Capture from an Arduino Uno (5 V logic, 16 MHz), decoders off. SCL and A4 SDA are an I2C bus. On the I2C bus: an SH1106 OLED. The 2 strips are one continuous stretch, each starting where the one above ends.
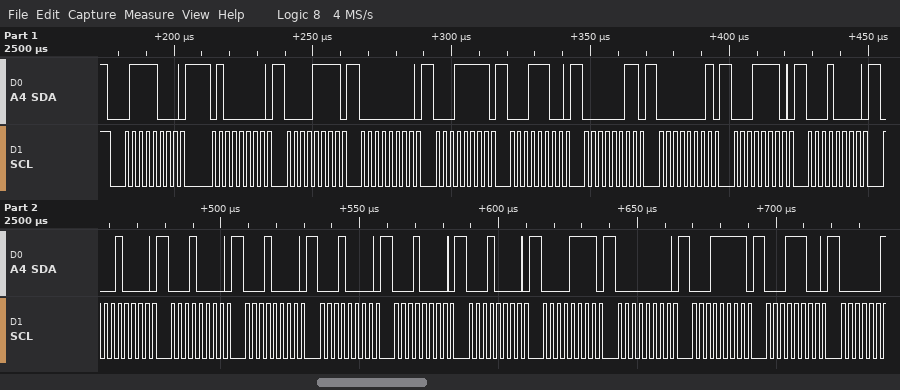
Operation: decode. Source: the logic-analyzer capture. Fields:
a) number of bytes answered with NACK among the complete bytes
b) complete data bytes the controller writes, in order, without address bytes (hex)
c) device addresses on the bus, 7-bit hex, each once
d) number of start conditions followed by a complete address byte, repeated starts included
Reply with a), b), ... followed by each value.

a) 0
b) 40 0F 00 1F 1C 03 01 1E 10 10 10 10 10 10 10 0F 00 1F 1C
c) 0x3C
d) 1
